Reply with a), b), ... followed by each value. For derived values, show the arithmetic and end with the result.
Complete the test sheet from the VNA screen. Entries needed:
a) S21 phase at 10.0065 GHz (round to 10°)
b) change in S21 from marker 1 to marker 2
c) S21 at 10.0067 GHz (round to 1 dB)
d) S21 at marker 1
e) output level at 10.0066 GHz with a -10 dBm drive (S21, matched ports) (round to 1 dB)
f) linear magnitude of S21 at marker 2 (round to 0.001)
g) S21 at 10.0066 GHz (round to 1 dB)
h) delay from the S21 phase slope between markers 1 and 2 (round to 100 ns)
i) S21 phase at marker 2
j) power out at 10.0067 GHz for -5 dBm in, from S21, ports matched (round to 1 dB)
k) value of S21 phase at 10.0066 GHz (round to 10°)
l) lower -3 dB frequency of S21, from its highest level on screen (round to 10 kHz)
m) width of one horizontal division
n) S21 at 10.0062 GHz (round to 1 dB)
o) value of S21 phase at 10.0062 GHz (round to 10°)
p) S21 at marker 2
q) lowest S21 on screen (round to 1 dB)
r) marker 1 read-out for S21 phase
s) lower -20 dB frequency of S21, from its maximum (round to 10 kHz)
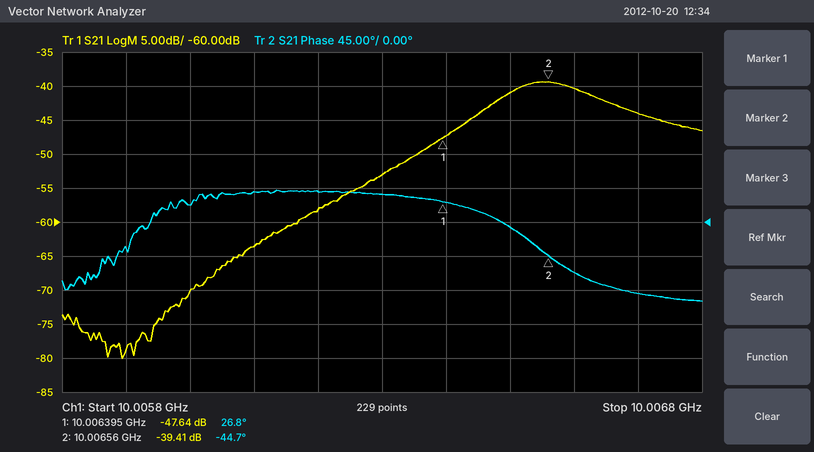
a) -10°
b) -39.41 − (-47.64) = 8.23 dB
c) -44 dB
d) -47.64 dB
e) -10 dBm + (-40 dB) = -50 dBm
f) 10^(-39.41/20) ≈ 0.011
g) -40 dB
h) −(-44.7° − (26.8°))/(360° × 165 kHz) ≈ 1.2 µs
i) -44.7°
j) -5 dBm + (-44 dB) = -49 dBm
k) -70°
l) 10.00648 GHz
m) 100 kHz
n) -58 dB
o) 40°
p) -39.41 dB
q) -80 dB
r) 26.8°
s) 10.00618 GHz
